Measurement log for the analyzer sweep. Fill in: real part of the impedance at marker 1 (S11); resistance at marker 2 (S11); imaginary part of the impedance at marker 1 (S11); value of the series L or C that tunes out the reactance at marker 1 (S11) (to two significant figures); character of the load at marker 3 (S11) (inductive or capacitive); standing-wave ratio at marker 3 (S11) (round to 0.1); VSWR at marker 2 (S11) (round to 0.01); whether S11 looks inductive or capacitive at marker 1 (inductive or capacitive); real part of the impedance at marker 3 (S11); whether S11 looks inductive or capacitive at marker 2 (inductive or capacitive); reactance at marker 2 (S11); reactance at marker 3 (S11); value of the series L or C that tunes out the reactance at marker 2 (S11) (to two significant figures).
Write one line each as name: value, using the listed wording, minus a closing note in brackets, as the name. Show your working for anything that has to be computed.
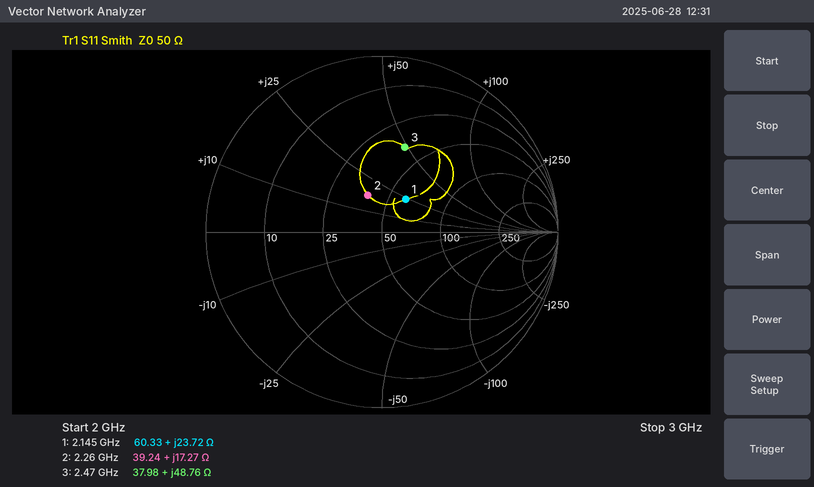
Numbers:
real part of the impedance at marker 1: 60.33 Ω
resistance at marker 2: 39.24 Ω
imaginary part of the impedance at marker 1: +23.72 Ω
value of the series L or C that tunes out the reactance at marker 1 (S11): C = 1/(2π × 2.145 GHz × 23.72 Ω) ≈ 3.1 pF
character of the load at marker 3 (S11): inductive
standing-wave ratio at marker 3 (S11): 3.0
VSWR at marker 2 (S11): 1.58
whether S11 looks inductive or capacitive at marker 1: inductive
real part of the impedance at marker 3: 37.98 Ω
whether S11 looks inductive or capacitive at marker 2: inductive
reactance at marker 2: +17.27 Ω
reactance at marker 3: +48.76 Ω
value of the series L or C that tunes out the reactance at marker 2 (S11): C = 1/(2π × 2.26 GHz × 17.27 Ω) ≈ 4.1 pF
